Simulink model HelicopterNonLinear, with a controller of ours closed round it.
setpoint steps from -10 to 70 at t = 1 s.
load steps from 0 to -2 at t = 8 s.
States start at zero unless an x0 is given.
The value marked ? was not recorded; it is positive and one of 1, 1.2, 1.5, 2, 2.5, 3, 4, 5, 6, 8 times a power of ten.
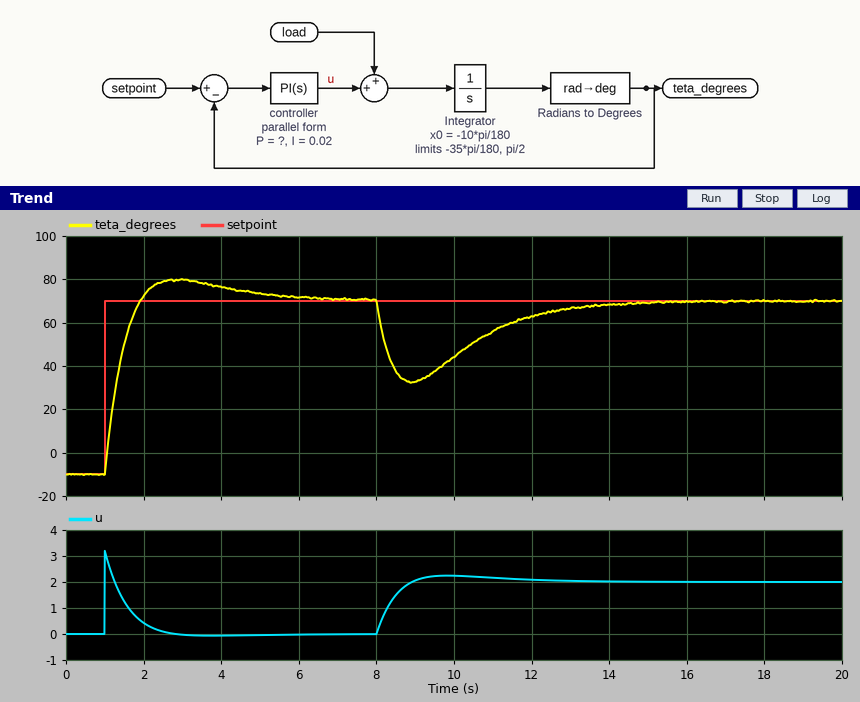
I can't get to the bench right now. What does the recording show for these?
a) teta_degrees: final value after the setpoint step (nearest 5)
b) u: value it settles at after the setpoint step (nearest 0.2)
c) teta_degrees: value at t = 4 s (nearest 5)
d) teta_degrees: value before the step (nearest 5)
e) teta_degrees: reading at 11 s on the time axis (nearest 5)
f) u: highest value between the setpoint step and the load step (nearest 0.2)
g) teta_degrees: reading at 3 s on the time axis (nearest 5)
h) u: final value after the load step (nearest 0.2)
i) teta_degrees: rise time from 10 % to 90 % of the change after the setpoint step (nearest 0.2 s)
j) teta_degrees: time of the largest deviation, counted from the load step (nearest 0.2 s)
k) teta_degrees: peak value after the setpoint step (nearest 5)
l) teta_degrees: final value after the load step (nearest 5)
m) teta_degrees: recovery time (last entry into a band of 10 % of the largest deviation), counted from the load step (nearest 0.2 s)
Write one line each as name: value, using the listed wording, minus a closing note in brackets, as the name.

teta_degrees: final value after the setpoint step: 70
u: value it settles at after the setpoint step: 0.0
teta_degrees: value at t = 4 s: 75
teta_degrees: value before the step: -10
teta_degrees: reading at 11 s on the time axis: 55
u: highest value between the setpoint step and the load step: 3.2
teta_degrees: reading at 3 s on the time axis: 80
u: final value after the load step: 2.0
teta_degrees: rise time from 10 % to 90 % of the change after the setpoint step: 0.6 s
teta_degrees: time of the largest deviation, counted from the load step: 1.0 s
teta_degrees: peak value after the setpoint step: 80
teta_degrees: final value after the load step: 70
teta_degrees: recovery time (last entry into a band of 10 % of the largest deviation), counted from the load step: 4.8 s
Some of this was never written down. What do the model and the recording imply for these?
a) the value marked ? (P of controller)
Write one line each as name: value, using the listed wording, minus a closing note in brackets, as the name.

the value marked ?: 0.04
